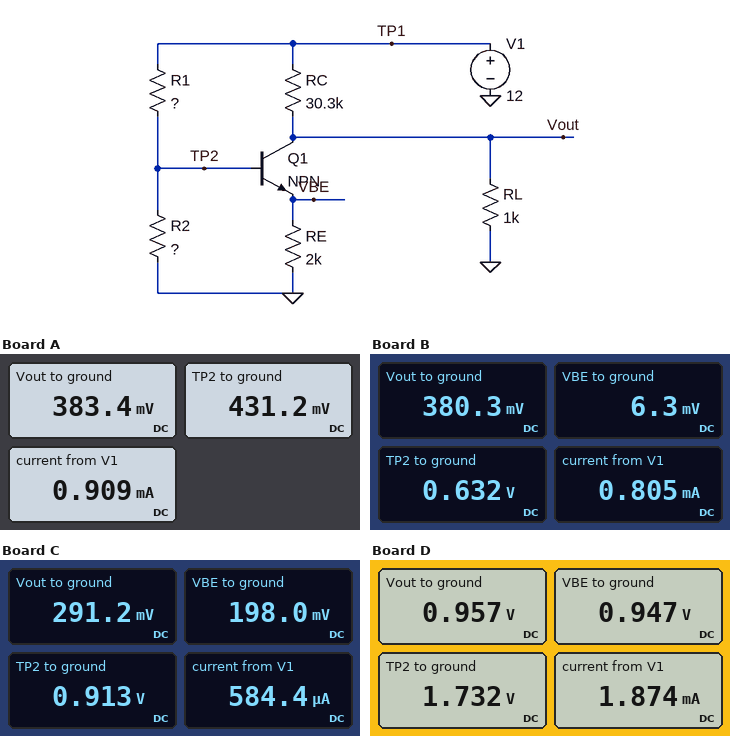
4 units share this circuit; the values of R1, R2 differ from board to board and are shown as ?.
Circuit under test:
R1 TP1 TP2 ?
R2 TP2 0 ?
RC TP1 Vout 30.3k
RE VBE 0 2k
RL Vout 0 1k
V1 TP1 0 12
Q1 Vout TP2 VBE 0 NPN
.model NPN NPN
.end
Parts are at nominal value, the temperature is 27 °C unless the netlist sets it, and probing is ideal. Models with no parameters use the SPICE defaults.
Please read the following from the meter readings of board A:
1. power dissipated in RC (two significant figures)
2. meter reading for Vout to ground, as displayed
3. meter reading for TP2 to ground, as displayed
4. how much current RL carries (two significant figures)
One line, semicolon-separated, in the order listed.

4.5 mW; 383.4 mV; 431.2 mV; 380 µA
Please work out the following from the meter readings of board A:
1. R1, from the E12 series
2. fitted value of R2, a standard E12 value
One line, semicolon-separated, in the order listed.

22 kΩ; 820 Ω
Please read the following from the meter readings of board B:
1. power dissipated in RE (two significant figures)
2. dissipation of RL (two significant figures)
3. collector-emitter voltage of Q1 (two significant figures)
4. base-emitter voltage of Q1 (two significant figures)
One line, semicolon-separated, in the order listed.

20 nW; 140 µW; 370 mV; 630 mV
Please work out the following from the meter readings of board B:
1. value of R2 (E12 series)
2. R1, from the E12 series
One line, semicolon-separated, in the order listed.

1.5 kΩ; 27 kΩ
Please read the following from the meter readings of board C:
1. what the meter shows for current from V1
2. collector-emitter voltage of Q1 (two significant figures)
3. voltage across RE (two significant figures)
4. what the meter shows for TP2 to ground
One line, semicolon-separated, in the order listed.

584.4 µA; 93 mV; 200 mV; 0.913 V
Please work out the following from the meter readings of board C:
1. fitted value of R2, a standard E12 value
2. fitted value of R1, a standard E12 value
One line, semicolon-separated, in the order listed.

4.7 kΩ; 56 kΩ
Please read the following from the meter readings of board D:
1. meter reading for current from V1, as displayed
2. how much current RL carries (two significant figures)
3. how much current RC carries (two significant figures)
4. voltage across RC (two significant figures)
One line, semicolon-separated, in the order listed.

1.874 mA; 960 µA; 360 µA; 11 V
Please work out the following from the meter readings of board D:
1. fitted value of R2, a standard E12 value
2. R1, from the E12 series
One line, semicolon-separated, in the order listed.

3.9 kΩ; 6.8 kΩ
